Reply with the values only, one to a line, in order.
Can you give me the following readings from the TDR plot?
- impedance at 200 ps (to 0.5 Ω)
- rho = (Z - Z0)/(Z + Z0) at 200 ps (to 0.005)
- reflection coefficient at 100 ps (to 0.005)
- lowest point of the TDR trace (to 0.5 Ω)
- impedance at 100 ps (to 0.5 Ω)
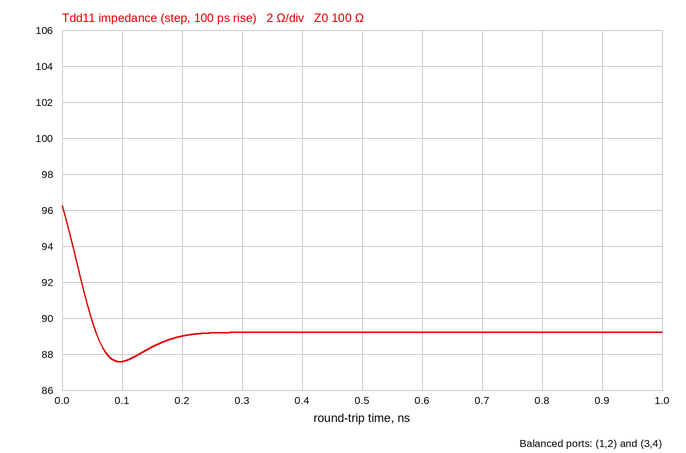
89.0 Ω
-0.060
-0.065
87.5 Ω
87.5 Ω
